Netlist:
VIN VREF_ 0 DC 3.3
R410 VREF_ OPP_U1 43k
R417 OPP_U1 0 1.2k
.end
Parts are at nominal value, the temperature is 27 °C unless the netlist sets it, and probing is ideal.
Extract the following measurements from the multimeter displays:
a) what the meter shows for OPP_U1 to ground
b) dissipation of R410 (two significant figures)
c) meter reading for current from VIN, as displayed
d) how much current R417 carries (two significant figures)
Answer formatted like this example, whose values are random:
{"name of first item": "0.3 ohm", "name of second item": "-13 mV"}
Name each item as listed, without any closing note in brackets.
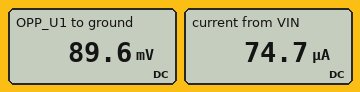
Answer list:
{"what the meter shows for OPP_U1 to ground": "89.6 mV", "dissipation of R410": "240 µW", "meter reading for current from VIN, as displayed": "74.7 µA", "how much current R417 carries": "75 µA"}
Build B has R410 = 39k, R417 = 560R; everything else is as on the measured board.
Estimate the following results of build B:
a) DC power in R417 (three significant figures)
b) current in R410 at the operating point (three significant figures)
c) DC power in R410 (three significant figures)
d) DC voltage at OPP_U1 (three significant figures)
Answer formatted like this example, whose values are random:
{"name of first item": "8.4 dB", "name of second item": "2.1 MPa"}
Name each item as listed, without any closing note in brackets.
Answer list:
{"DC power in R417": "3.90 µW", "current in R410 at the operating point": "83.4 µA", "DC power in R410": "271 µW", "DC voltage at OPP_U1": "46.7 mV"}
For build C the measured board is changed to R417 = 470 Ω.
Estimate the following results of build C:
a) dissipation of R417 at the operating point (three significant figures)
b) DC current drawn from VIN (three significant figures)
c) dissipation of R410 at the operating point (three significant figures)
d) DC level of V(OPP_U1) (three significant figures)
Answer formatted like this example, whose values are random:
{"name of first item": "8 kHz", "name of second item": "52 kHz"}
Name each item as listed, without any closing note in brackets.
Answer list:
{"dissipation of R417 at the operating point": "2.71 µW", "DC current drawn from VIN": "75.9 µA", "dissipation of R410 at the operating point": "248 µW", "DC level of V(OPP_U1)": "35.7 mV"}
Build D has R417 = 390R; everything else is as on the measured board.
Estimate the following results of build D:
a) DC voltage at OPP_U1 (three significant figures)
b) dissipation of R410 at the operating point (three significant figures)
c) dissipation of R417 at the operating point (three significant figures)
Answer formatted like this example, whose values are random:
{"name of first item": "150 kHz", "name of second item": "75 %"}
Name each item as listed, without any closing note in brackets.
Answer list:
{"DC voltage at OPP_U1": "29.7 mV", "dissipation of R410 at the operating point": "249 µW", "dissipation of R417 at the operating point": "2.26 µW"}
